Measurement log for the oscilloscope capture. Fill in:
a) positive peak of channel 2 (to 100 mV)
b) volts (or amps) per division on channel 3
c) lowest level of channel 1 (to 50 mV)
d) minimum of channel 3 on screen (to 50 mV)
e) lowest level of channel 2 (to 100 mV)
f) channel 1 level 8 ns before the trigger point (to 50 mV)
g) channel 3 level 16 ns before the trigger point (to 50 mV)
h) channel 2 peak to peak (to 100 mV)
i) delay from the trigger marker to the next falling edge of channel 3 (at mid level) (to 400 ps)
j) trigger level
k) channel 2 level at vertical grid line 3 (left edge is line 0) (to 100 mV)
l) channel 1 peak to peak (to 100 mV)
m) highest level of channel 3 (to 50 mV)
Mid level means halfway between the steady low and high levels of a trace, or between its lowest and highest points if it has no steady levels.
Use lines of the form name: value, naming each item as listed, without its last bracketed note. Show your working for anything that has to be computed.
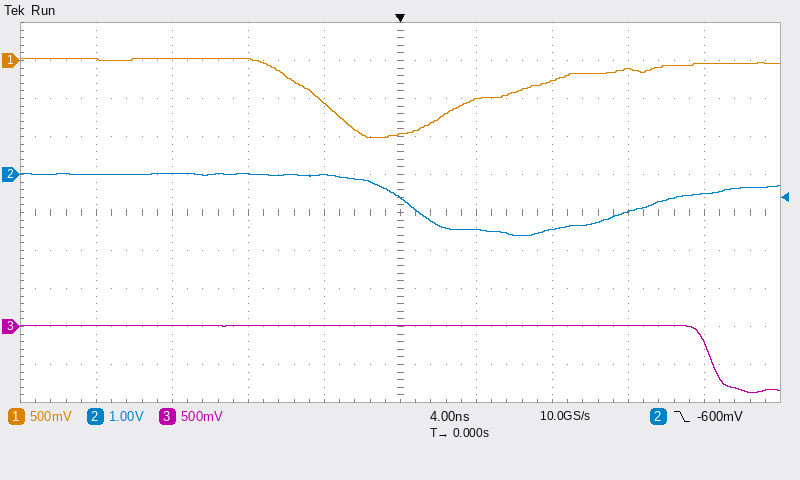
positive peak of channel 2: 0.0 V
volts (or amps) per division on channel 3: 500 mV
lowest level of channel 1: -1.00 V
minimum of channel 3 on screen: -850 mV
lowest level of channel 2: -1.6 V
channel 1 level 8 ns before the trigger point: 0 mV
channel 3 level 16 ns before the trigger point: 0 mV
channel 2 peak to peak: 0.0 V − (-1.6 V) = 1.6 V
delay from the trigger marker to the next falling edge of channel 3 (at mid level): 16.4 ns
trigger level: -600 mV
channel 2 level at vertical grid line 3 (left edge is line 0): 0.0 V
channel 1 peak to peak: 1.00 V
highest level of channel 3: 0 mV
